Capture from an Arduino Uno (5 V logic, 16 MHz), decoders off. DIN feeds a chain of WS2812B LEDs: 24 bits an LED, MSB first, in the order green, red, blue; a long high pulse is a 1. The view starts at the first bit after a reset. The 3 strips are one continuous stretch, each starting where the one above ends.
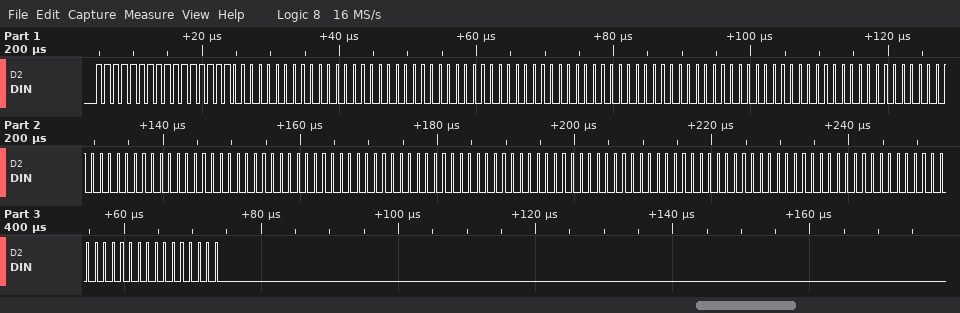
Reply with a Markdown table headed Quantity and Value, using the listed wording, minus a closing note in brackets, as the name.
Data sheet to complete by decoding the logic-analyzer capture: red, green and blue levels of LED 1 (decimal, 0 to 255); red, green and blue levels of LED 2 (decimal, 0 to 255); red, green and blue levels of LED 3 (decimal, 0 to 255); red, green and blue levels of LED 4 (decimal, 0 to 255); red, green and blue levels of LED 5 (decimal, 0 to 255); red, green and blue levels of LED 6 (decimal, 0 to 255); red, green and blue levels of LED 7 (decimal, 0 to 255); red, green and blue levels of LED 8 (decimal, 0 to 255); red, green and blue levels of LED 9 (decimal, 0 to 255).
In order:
| Quantity | Value |
|---|---|
| red, green and blue levels of LED 1 | 255, 255, 0 |
| red, green and blue levels of LED 2 | 0, 0, 0 |
| red, green and blue levels of LED 3 | 0, 0, 0 |
| red, green and blue levels of LED 4 | 0, 0, 0 |
| red, green and blue levels of LED 5 | 0, 0, 0 |
| red, green and blue levels of LED 6 | 0, 0, 0 |
| red, green and blue levels of LED 7 | 0, 0, 0 |
| red, green and blue levels of LED 8 | 0, 0, 0 |
| red, green and blue levels of LED 9 | 0, 0, 0 |
